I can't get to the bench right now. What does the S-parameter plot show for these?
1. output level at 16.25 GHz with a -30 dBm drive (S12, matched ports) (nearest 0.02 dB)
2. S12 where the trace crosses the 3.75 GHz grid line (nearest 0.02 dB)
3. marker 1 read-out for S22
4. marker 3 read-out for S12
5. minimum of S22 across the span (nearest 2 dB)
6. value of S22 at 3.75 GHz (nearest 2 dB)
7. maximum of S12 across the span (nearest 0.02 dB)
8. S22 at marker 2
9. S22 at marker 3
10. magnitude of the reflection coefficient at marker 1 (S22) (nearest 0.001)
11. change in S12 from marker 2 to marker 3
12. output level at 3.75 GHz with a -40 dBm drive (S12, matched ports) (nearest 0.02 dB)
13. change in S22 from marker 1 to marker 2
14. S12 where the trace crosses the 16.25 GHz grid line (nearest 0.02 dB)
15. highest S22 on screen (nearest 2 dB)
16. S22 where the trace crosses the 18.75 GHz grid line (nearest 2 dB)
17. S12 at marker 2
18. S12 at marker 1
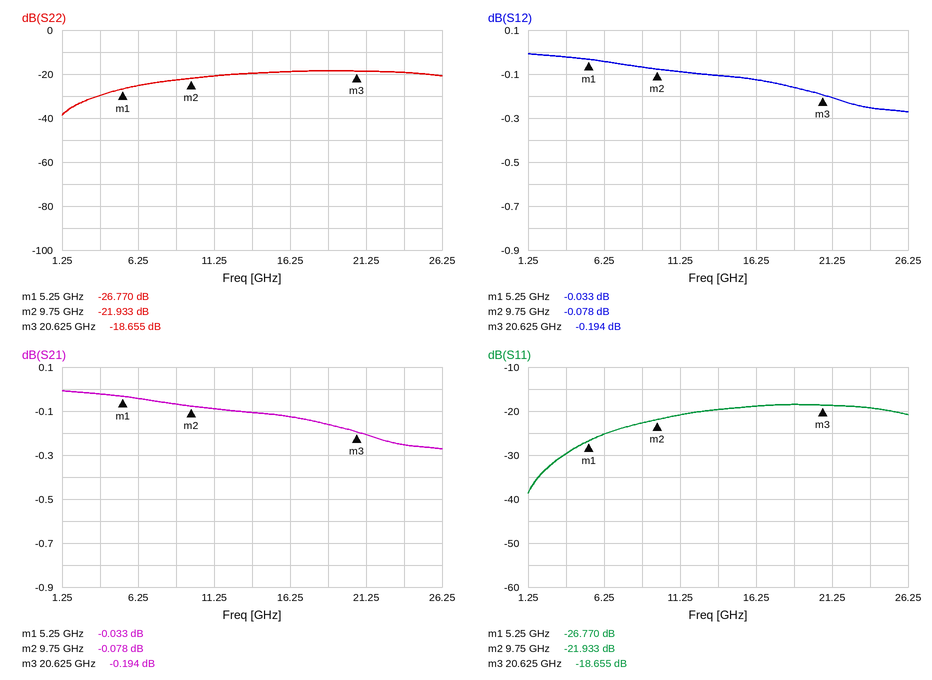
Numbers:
-30.12 dBm
-0.02 dB
-26.770 dB
-0.194 dB
-38 dB
-30 dB
0.00 dB
-21.933 dB
-18.655 dB
0.046
-0.116 dB
-40.02 dBm
4.837 dB
-0.12 dB
-18 dB
-18 dB
-0.078 dB
-0.033 dB
